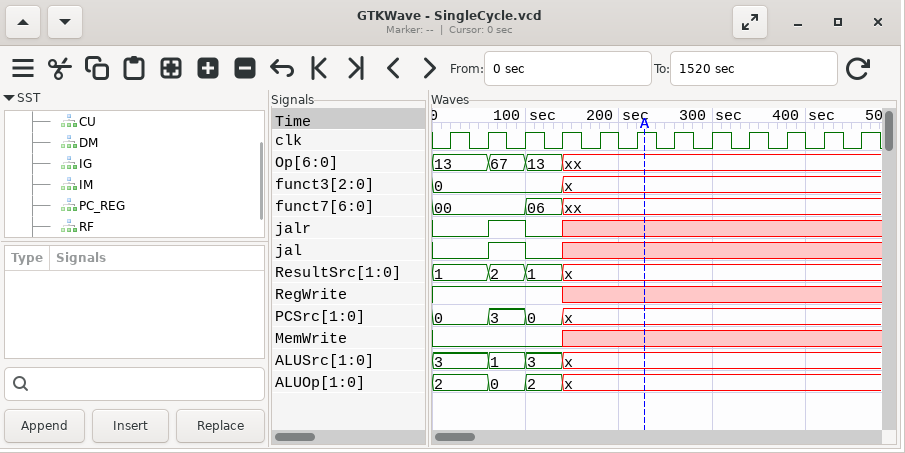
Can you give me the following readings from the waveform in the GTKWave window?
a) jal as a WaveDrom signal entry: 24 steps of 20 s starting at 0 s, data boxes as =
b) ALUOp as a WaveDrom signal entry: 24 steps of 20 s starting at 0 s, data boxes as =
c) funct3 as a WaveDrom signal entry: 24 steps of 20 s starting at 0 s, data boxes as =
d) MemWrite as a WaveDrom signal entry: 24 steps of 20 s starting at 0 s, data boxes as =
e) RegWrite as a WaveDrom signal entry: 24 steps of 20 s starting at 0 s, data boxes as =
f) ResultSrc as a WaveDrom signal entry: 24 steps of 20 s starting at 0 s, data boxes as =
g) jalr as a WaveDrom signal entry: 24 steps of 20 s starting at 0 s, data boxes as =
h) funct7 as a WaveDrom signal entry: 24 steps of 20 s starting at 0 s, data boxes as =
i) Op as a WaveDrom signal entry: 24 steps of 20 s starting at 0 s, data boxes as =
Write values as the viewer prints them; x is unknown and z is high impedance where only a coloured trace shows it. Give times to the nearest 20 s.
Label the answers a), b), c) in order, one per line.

a) {name: 'jal', wave: '0..1.0.x................'}
b) {name: 'ALUOp', wave: '=..=.=.x................', data: '2 0 2'}
c) {name: 'funct3', wave: '=......x................', data: '0'}
d) {name: 'MemWrite', wave: '0......x................'}
e) {name: 'RegWrite', wave: '1......x................'}
f) {name: 'ResultSrc', wave: '=..=.=.x................', data: '1 2 1'}
g) {name: 'jalr', wave: '0..1.0.x................'}
h) {name: 'funct7', wave: '=....=.x................', data: '00 06'}
i) {name: 'Op', wave: '=..=.=.x................', data: '13 67 13'}
